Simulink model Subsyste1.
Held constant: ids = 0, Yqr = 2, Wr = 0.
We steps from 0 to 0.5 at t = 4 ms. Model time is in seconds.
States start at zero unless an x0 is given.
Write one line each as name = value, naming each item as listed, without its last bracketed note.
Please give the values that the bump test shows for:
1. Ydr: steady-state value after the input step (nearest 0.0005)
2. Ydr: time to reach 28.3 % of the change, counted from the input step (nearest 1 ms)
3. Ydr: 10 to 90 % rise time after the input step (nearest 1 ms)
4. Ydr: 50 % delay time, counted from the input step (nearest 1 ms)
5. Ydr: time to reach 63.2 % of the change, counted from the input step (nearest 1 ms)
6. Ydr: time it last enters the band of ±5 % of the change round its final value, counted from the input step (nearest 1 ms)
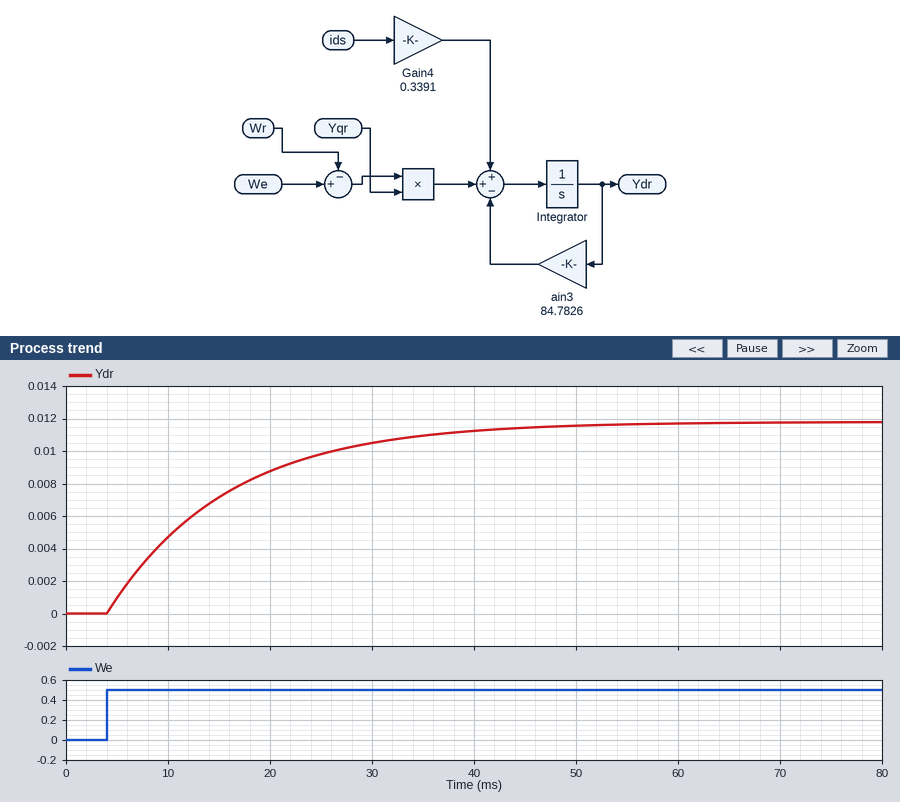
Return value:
Ydr: steady-state value after the input step = 0.0120
Ydr: time to reach 28.3 % of the change, counted from the input step = 4 ms
Ydr: 10 to 90 % rise time after the input step = 26 ms
Ydr: 50 % delay time, counted from the input step = 8 ms
Ydr: time to reach 63.2 % of the change, counted from the input step = 12 ms
Ydr: time it last enters the band of ±5 % of the change round its final value, counted from the input step = 35 ms
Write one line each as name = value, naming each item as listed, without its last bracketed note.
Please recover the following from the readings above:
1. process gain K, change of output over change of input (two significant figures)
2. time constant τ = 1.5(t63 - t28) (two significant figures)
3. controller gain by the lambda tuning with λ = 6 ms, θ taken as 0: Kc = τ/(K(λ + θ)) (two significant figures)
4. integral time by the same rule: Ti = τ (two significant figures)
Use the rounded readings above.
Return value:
process gain K, change of output over change of input = 0.024
time constant τ = 1.5(t63 - t28) = 12 ms
controller gain by the lambda tuning with λ = 6 ms, θ taken as 0: Kc = τ/(K(λ + θ)) = 83
integral time by the same rule: Ti = τ = 12 ms
